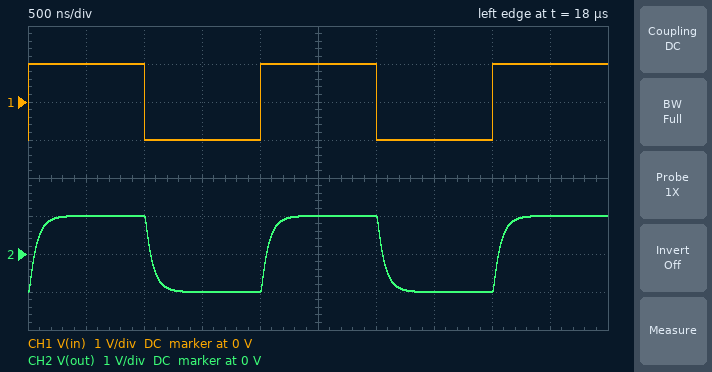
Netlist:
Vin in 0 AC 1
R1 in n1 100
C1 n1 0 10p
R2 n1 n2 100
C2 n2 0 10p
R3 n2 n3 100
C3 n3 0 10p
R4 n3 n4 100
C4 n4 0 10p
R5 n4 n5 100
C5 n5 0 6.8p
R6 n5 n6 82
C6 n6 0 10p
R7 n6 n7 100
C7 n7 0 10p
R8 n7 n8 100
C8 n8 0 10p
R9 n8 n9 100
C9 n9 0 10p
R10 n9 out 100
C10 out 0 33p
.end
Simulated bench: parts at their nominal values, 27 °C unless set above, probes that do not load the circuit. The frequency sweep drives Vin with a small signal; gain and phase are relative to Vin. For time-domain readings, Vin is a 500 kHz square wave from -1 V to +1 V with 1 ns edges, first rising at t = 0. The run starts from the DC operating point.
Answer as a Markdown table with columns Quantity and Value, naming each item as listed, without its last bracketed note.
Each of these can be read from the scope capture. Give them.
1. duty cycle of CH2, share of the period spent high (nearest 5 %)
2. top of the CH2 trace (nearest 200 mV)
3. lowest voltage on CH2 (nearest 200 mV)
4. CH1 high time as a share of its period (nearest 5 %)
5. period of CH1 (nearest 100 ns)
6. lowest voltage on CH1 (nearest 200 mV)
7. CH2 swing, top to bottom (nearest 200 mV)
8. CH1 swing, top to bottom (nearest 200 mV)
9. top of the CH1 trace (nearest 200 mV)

| Quantity | Value |
|---|---|
| duty cycle of CH2, share of the period spent high | 50 % |
| top of the CH2 trace | 1.0 V |
| lowest voltage on CH2 | -1.0 V |
| CH1 high time as a share of its period | 50 % |
| period of CH1 | 2.0 µs |
| lowest voltage on CH1 | -1.0 V |
| CH2 swing, top to bottom | 2.0 V |
| CH1 swing, top to bottom | 2.0 V |
| top of the CH1 trace | 1.0 V |
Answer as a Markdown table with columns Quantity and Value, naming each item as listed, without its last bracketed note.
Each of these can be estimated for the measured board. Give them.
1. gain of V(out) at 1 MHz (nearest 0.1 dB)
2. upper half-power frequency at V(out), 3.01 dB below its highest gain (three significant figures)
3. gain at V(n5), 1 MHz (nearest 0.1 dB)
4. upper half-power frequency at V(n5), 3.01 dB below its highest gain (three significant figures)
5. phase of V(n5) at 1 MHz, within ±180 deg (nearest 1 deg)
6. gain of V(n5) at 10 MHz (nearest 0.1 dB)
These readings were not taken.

| Quantity | Value |
|---|---|
| gain of V(out) at 1 MHz | -0.6 dB |
| upper half-power frequency at V(out), 3.01 dB below its highest gain | 2.49 MHz |
| gain at V(n5), 1 MHz | -0.6 dB |
| upper half-power frequency at V(n5), 3.01 dB below its highest gain | 2.85 MHz |
| phase of V(n5) at 1 MHz, within ±180 deg | -17 deg |
| gain of V(n5) at 10 MHz | -8.3 dB |
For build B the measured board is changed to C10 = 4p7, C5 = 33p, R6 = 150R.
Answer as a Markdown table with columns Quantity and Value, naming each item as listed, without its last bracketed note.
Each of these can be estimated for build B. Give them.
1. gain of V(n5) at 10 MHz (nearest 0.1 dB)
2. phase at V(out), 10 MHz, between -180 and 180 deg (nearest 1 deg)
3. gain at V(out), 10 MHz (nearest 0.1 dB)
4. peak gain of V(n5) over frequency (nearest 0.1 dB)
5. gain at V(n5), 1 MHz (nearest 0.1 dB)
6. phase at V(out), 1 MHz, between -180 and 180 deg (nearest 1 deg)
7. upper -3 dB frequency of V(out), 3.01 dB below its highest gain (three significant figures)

| Quantity | Value |
|---|---|
| gain of V(n5) at 10 MHz | -9.3 dB |
| phase at V(out), 10 MHz, between -180 and 180 deg | -115 deg |
| gain at V(out), 10 MHz | -11.3 dB |
| peak gain of V(n5) over frequency | 0 dB |
| gain at V(n5), 1 MHz | -0.4 dB |
| phase at V(out), 1 MHz, between -180 and 180 deg | -22 deg |
| upper -3 dB frequency of V(out), 3.01 dB below its highest gain | 3.04 MHz |
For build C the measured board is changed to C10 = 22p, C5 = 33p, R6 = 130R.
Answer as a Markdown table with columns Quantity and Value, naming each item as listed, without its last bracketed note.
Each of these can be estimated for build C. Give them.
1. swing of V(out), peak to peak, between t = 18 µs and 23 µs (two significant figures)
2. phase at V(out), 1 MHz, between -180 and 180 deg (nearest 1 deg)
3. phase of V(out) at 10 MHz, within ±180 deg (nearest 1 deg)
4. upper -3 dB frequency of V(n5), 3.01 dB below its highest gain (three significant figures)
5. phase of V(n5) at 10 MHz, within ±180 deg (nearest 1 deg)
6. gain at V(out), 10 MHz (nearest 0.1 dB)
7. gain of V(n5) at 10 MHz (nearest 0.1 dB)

| Quantity | Value |
|---|---|
| swing of V(out), peak to peak, between t = 18 µs and 23 µs | 2.0 V |
| phase at V(out), 1 MHz, between -180 and 180 deg | -28 deg |
| phase of V(out) at 10 MHz, within ±180 deg | -127 deg |
| upper -3 dB frequency of V(n5), 3.01 dB below its highest gain | 2.62 MHz |
| phase of V(n5) at 10 MHz, within ±180 deg | -64 deg |
| gain at V(out), 10 MHz | -13.7 dB |
| gain of V(n5) at 10 MHz | -9.7 dB |
